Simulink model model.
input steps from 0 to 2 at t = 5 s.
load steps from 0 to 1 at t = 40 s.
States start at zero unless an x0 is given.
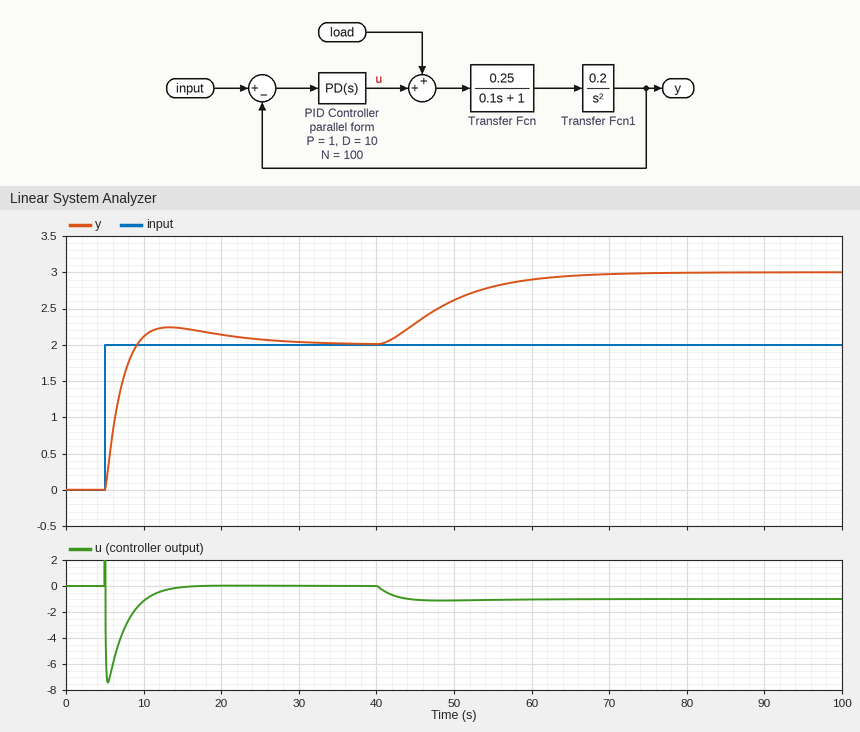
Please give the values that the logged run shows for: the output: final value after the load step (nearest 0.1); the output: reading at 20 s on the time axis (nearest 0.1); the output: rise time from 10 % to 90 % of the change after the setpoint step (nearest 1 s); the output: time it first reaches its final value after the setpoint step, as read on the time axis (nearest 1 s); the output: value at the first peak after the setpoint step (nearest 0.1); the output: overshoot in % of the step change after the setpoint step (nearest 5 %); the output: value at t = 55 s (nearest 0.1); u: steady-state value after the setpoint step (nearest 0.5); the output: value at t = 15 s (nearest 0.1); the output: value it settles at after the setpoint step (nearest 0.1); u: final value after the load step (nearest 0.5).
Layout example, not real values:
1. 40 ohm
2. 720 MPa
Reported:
1. 3.0
2. 2.1
3. 3 s
4. 9 s
5. 2.2
6. 10 %
7. 2.8
8. 0.0
9. 2.2
10. 2.0
11. -1.0
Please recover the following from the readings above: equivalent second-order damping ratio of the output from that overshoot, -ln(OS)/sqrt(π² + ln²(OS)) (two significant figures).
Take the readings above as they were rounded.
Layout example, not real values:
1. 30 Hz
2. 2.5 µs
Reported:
1. 0.59
